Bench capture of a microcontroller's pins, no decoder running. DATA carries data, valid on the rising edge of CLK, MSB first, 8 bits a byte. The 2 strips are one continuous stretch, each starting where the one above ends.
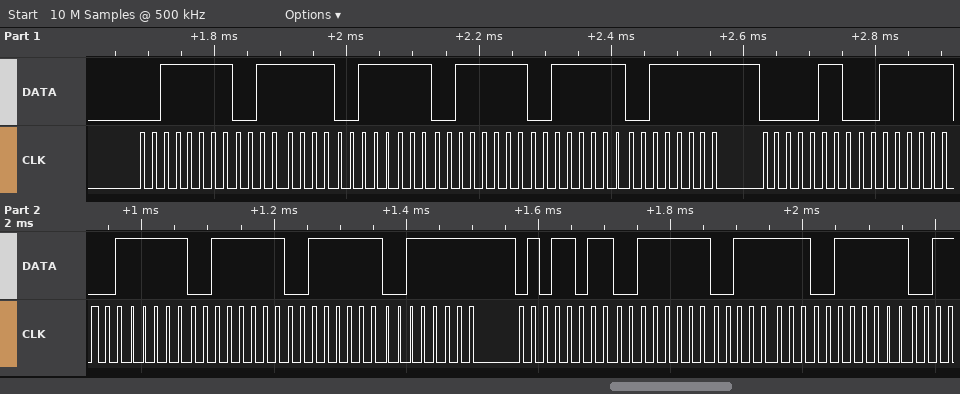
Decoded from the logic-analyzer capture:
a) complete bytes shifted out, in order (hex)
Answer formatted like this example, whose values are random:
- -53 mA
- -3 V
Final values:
- 0x3F 0x3F 0x3F 0x3F 0x3F 0x3F 0x06 0x3F 0x3F 0x3F 0x3F 0x3F 0x5B 0x3F 0x3F 0x3F
